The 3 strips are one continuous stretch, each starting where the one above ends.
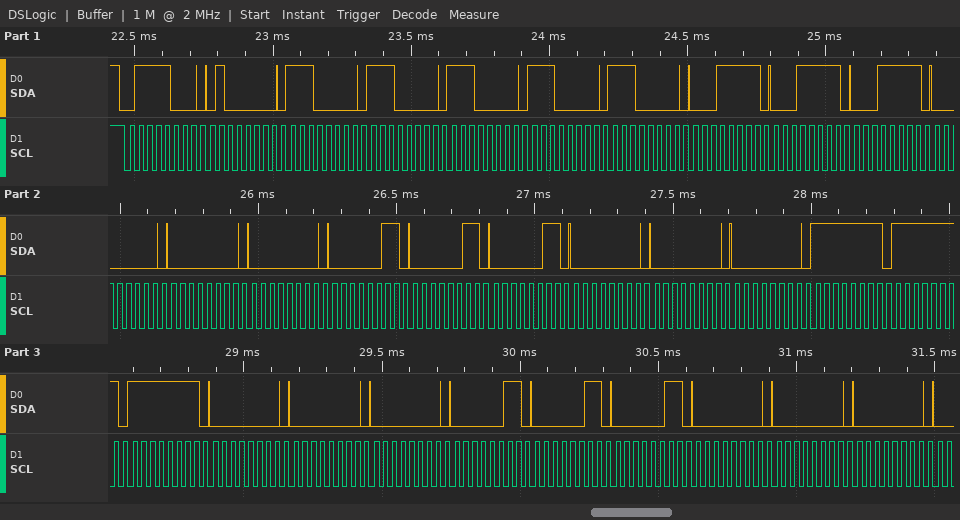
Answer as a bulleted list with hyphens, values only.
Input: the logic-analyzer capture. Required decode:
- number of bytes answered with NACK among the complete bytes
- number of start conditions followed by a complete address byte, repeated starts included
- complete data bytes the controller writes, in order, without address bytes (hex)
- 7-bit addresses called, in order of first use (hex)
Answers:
- 0
- 1
- 40 E0 E0 E0 E0 E0 1F 1F 1F 00 00 00 03 03 03 00 00 00 FF FF FF 00 00 00 03 03 03 00 00 00
- 0x3C
